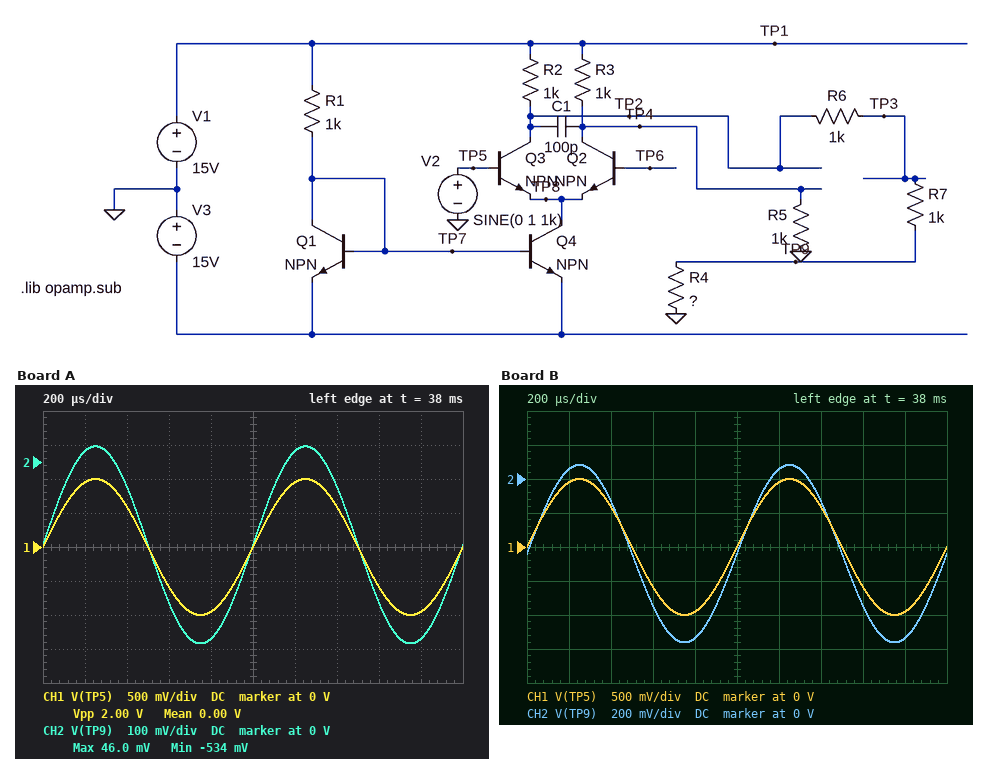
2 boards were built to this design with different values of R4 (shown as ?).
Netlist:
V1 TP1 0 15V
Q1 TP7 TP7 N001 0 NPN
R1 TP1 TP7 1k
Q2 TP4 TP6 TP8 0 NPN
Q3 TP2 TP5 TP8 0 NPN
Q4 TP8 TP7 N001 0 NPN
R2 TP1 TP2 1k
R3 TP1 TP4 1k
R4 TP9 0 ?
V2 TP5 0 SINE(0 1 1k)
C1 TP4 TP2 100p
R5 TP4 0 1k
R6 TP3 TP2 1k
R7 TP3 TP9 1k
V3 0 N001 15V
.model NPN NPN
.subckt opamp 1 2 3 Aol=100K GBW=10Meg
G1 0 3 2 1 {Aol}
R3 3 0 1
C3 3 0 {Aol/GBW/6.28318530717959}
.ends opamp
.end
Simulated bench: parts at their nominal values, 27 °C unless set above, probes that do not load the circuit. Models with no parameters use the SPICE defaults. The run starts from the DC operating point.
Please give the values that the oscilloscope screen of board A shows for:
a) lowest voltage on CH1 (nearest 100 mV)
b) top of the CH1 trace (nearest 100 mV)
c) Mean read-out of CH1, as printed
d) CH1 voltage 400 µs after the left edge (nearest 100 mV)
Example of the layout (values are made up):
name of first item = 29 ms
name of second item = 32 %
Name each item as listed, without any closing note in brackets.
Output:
lowest voltage on CH1 = -1.0 V
top of the CH1 trace = 1.0 V
Mean read-out of CH1, as printed = 0.00 V
CH1 voltage 400 µs after the left edge = 600 mV
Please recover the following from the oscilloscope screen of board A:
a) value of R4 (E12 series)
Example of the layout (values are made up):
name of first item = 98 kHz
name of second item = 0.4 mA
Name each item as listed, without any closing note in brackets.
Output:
value of R4 = 820 Ω
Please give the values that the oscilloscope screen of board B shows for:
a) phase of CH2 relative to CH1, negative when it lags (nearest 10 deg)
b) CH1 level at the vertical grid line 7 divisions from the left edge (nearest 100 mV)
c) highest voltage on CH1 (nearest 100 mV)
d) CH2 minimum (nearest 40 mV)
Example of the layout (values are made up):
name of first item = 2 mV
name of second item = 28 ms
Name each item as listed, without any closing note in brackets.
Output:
phase of CH2 relative to CH1, negative when it lags = 0 deg
CH1 level at the vertical grid line 7 divisions from the left edge = 600 mV
highest voltage on CH1 = 1.0 V
CH2 minimum = -960 mV
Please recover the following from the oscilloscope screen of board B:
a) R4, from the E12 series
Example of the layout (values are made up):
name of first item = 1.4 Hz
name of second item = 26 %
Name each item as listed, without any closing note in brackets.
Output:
R4, from the E12 series = 2.2 kΩ
